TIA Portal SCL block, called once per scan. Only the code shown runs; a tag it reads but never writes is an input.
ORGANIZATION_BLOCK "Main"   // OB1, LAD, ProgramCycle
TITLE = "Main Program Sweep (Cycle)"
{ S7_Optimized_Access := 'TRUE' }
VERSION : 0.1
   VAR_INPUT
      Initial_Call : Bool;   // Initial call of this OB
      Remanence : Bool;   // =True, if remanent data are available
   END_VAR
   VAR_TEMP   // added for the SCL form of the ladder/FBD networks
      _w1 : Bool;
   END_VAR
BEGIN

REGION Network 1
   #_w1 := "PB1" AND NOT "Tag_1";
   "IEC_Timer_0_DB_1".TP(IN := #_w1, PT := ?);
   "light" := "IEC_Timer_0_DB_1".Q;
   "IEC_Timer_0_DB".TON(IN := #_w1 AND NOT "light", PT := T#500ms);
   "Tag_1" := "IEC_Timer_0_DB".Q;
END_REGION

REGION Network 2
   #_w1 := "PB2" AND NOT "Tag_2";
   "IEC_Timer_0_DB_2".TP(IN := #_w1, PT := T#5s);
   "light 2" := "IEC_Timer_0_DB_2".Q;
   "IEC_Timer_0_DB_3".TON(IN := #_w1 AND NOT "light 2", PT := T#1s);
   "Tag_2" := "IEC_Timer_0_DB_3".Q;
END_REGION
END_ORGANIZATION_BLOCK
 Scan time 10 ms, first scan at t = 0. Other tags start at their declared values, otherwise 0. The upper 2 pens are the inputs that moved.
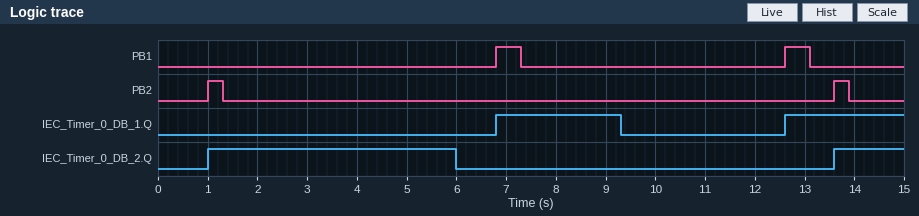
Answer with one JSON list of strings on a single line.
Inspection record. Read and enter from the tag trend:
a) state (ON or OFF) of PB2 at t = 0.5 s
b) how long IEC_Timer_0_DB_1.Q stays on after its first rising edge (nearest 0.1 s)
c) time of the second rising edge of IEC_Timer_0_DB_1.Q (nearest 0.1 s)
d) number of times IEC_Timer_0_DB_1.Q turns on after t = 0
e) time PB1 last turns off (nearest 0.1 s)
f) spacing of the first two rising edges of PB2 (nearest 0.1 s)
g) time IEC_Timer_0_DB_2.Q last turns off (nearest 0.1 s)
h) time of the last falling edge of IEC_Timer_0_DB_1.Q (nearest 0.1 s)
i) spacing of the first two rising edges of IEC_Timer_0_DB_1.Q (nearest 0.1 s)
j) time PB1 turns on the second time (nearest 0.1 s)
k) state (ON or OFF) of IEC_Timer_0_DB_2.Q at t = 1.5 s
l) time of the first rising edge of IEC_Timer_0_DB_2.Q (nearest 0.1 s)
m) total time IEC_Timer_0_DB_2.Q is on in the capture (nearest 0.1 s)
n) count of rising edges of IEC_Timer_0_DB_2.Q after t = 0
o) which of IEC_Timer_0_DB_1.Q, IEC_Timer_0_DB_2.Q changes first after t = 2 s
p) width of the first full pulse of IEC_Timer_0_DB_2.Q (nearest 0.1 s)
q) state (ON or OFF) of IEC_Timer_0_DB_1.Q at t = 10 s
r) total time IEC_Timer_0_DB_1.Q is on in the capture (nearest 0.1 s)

["OFF", "2.5 s", "12.6 s", "2", "13.1 s", "12.6 s", "6.0 s", "9.3 s", "5.8 s", "12.6 s", "ON", "1.0 s", "6.4 s", "2", "IEC_Timer_0_DB_2.Q", "5.0 s", "OFF", "4.9 s"]
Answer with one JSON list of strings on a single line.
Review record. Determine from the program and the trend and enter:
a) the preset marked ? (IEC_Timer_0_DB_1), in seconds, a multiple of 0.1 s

["2.5 s"]
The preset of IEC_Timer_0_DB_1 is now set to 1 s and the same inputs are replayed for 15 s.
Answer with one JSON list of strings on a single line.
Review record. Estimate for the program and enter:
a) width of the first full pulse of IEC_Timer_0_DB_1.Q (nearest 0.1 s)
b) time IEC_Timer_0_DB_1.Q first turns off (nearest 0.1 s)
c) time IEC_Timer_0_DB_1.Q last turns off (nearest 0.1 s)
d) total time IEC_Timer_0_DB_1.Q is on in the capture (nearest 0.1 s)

["1.0 s", "7.8 s", "13.6 s", "2.0 s"]
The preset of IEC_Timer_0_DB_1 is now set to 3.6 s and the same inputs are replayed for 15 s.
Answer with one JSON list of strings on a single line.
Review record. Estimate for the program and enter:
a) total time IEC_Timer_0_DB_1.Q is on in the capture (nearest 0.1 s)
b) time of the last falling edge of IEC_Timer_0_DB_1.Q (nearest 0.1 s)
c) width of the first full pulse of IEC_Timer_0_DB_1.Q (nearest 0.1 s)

["6.0 s", "10.4 s", "3.6 s"]
